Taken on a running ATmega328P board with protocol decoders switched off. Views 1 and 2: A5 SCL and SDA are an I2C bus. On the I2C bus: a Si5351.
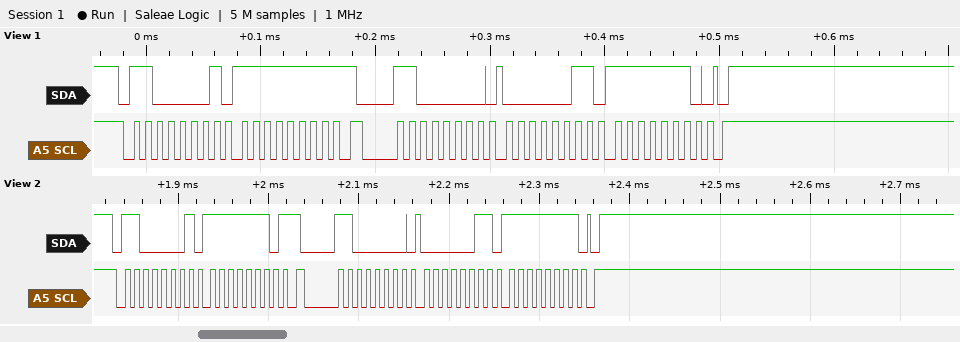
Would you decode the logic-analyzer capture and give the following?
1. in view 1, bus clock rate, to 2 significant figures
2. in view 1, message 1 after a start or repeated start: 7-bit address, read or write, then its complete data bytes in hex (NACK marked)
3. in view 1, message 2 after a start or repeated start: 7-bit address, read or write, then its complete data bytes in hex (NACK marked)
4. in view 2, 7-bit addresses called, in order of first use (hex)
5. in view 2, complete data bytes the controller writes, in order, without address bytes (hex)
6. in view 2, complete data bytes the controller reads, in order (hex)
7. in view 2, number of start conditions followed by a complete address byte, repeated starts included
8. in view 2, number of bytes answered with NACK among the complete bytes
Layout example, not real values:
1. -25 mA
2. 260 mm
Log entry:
1. 100 kHz
2. 0x60 read: FF NACK
3. 0x60 write: 03 FE
4. 0x60
5. 03 FF
6. FE
7. 2
8. 1
